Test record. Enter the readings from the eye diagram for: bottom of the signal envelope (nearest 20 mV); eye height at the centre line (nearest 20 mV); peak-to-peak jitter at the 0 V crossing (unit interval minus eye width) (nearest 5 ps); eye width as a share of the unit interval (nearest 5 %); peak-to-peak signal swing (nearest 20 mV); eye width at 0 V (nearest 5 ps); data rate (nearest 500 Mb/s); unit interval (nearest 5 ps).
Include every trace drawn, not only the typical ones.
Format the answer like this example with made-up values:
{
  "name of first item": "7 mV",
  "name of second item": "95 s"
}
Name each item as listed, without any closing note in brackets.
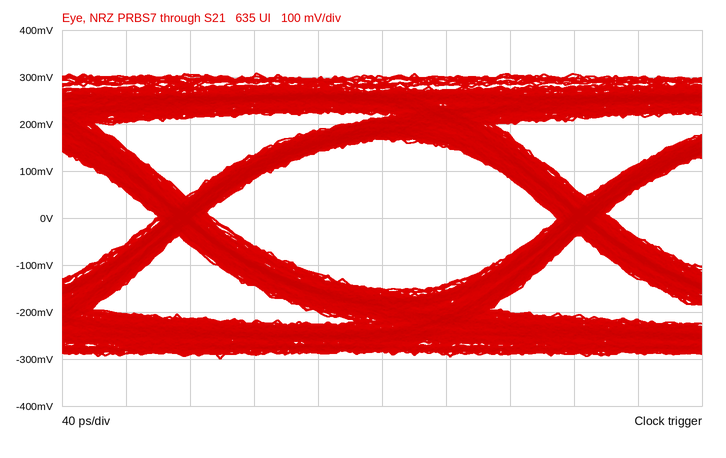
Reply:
{
  "bottom of the signal envelope": "-300 mV",
  "eye height at the centre line": "320 mV",
  "peak-to-peak jitter at the 0 V crossing (unit interval minus eye width)": "35 ps",
  "eye width as a share of the unit interval": "85 %",
  "peak-to-peak signal swing": "600 mV",
  "eye width at 0 V": "215 ps",
  "data rate": "4.0 Gb/s",
  "unit interval": "250 ps"
}
